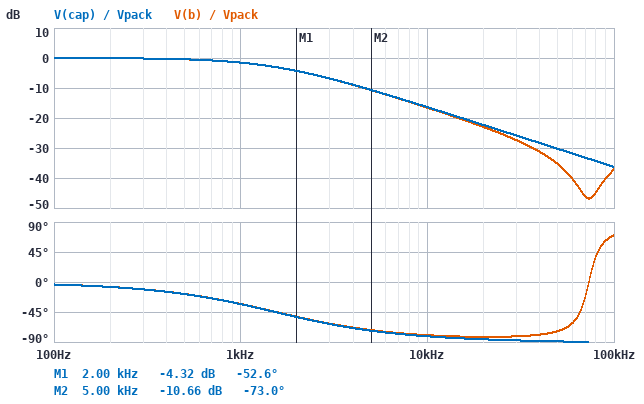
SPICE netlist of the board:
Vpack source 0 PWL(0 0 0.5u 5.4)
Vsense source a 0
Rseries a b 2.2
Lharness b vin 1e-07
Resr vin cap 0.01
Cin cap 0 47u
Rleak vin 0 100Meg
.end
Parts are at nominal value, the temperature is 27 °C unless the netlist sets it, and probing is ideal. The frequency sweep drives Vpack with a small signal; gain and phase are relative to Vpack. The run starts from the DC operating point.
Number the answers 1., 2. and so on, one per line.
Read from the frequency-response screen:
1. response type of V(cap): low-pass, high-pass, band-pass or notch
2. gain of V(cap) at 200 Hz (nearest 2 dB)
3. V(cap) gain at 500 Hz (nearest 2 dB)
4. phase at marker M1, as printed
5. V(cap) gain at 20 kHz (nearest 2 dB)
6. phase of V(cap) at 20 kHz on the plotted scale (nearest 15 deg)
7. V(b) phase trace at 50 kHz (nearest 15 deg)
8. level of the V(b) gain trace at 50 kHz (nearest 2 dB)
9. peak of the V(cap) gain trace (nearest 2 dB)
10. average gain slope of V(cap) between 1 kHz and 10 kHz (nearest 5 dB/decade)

1. low-pass
2. 0 dB
3. 0 dB
4. -52.6 deg
5. -22 dB
6. -90 deg
7. -75 deg
8. -36 dB
9. 0 dB
10. -15 dB/decade
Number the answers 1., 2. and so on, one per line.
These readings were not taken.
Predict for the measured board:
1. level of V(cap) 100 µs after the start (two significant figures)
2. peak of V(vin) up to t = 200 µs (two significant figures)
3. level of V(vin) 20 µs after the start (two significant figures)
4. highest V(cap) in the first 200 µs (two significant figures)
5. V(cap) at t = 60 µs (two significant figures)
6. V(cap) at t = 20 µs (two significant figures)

1. 3.3 V
2. 4.6 V
3. 950 mV
4. 4.6 V
5. 2.4 V
6. 930 mV
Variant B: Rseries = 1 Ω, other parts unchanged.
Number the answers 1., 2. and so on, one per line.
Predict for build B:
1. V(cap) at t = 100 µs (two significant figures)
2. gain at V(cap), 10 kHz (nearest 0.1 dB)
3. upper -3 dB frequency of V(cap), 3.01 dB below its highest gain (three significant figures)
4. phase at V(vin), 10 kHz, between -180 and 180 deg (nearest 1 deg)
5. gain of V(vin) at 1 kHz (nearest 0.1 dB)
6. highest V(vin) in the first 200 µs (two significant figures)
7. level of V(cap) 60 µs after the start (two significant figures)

1. 4.7 V
2. -9.9 dB
3. 3.36 kHz
4. -70 deg
5. -0.4 dB
6. 5.3 V
7. 3.9 V
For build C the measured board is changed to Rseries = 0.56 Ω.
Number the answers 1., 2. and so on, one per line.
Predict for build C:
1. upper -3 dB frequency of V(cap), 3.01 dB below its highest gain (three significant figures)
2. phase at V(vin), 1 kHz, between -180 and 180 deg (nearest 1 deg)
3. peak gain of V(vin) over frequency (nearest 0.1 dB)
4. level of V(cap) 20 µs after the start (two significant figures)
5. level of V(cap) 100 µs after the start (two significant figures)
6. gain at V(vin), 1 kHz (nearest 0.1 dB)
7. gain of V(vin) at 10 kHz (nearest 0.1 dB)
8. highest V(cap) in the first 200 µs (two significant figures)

1. 5.98 kHz
2. -9 deg
3. 0 dB
4. 2.8 V
5. 5.3 V
6. -0.1 dB
7. -5.8 dB
8. 5.4 V
